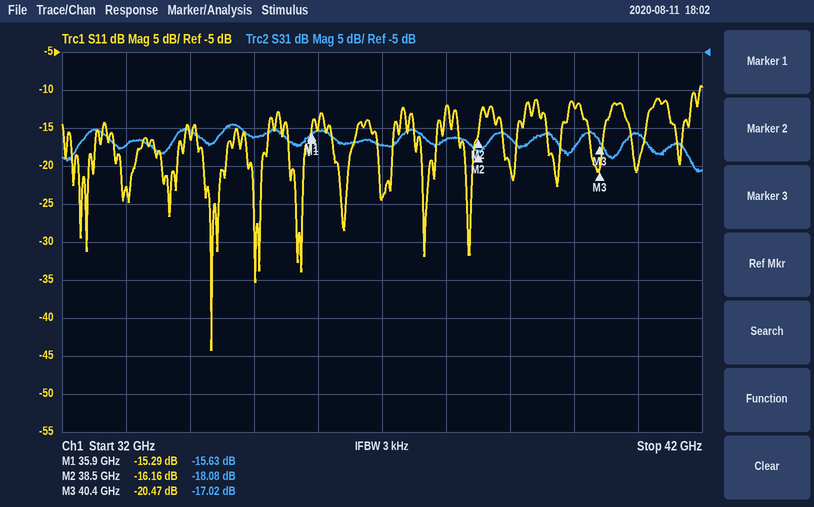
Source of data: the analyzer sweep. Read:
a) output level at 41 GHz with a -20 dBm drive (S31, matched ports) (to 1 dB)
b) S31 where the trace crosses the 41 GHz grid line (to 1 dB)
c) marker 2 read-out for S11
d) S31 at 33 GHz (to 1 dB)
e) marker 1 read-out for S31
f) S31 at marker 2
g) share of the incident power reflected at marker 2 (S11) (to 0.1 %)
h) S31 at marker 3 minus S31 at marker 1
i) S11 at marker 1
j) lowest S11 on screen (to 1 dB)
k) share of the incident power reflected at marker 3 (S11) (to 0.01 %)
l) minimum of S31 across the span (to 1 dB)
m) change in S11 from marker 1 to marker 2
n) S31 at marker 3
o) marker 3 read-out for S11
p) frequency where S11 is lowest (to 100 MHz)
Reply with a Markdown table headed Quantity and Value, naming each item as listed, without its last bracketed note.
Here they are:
| Quantity | Value |
|---|---|
| output level at 41 GHz with a -20 dBm drive (S31, matched ports) | -36 dBm |
| S31 where the trace crosses the 41 GHz grid line | -16 dB |
| marker 2 read-out for S11 | -16.16 dB |
| S31 at 33 GHz | -17 dB |
| marker 1 read-out for S31 | -15.63 dB |
| S31 at marker 2 | -18.08 dB |
| share of the incident power reflected at marker 2 (S11) | 2.4 % |
| S31 at marker 3 minus S31 at marker 1 | -1.39 dB |
| S11 at marker 1 | -15.29 dB |
| lowest S11 on screen | -44 dB |
| share of the incident power reflected at marker 3 (S11) | 0.90 % |
| minimum of S31 across the span | -21 dB |
| change in S11 from marker 1 to marker 2 | -0.87 dB |
| S31 at marker 3 | -17.02 dB |
| marker 3 read-out for S11 | -20.47 dB |
| frequency where S11 is lowest | 34.3 GHz |
